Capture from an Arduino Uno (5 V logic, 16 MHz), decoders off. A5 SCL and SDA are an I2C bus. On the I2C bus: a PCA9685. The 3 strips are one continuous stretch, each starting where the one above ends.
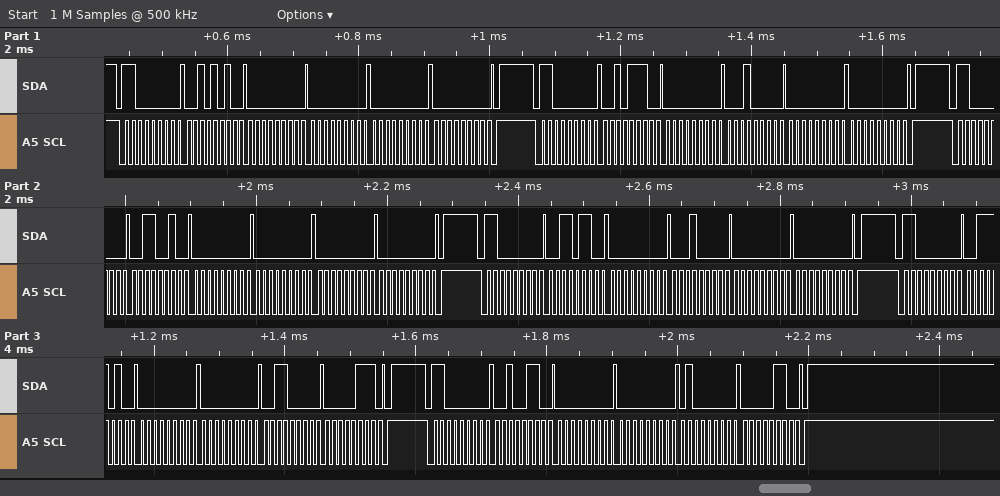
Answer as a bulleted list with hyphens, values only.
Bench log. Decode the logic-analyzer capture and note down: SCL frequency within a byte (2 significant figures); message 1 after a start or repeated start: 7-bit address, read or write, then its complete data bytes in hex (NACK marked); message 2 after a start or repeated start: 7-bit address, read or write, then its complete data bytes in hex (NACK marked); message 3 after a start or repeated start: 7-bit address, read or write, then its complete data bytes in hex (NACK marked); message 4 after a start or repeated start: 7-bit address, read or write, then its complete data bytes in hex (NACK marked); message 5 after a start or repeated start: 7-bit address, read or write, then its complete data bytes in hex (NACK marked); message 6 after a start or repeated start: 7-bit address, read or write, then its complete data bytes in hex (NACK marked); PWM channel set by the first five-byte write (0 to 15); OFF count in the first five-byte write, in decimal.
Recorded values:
- 100 kHz
- 0x60 write: 2A 00 00 00 00
- 0x60 write: 2E 00 10 00 00
- 0x60 write: 32 00 00 00 00
- 0x60 write: 36 00 10 00 00
- 0x60 write: 3A 00 00 30 07
- 0x60 write: 26 00 00 40 06
- 9
- 0
